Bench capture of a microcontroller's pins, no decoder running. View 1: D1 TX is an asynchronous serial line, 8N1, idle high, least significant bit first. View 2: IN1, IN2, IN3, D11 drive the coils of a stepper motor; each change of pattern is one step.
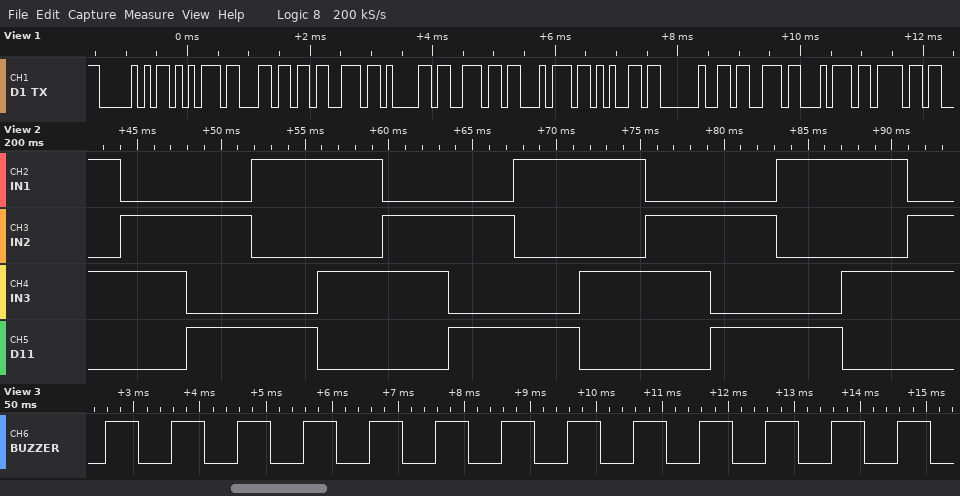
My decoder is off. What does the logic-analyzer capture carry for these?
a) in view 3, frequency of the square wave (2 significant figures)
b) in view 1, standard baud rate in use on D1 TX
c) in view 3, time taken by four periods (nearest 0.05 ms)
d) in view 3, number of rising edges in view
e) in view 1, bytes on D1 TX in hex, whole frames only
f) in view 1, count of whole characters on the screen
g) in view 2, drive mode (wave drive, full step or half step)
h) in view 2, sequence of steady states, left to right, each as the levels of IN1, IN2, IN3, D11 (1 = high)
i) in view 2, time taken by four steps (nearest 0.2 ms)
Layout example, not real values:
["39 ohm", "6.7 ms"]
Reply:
["1.00 kHz", "9600 baud", "4.00 ms", "13", "0x50 0x75 0x6C 0x73 0x61 0x6E 0x74 0x65 0x20 0x73 0x74 0x6F", "12", "full step", "1010 0110 0101 1001 1010 0110 0101 1001 1010 0110 0101 1001 1010 0110", "15.6 ms"]
